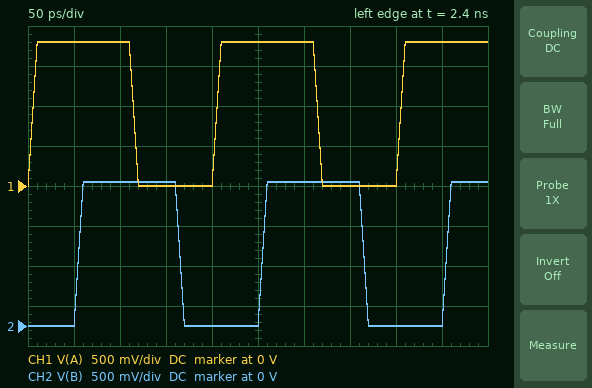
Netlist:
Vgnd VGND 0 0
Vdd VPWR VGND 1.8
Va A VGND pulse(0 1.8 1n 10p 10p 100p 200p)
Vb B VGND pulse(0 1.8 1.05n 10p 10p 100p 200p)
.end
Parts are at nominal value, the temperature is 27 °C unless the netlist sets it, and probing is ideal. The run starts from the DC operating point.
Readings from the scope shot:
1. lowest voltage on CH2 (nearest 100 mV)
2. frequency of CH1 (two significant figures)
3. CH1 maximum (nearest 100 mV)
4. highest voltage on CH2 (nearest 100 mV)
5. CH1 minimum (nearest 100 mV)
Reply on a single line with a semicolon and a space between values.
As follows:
0 V; 5.0 GHz; 1.8 V; 1.8 V; 0 V
